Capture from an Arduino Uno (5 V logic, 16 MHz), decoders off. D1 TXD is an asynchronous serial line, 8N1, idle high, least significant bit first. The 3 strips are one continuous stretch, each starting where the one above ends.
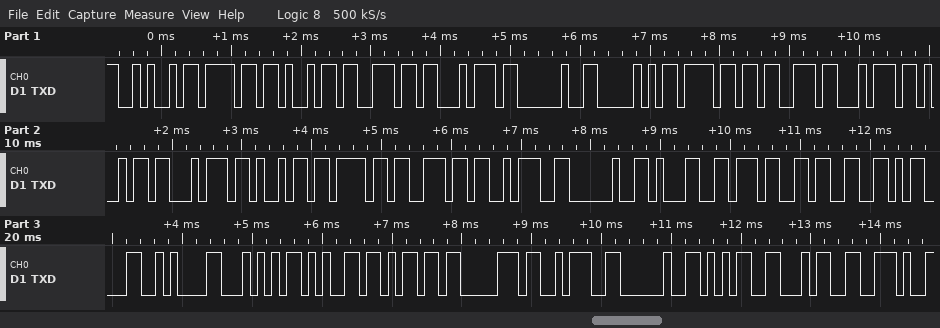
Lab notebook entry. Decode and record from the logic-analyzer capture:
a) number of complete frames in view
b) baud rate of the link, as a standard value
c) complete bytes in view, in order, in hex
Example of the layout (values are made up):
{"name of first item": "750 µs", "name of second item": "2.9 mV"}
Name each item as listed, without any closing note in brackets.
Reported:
{"number of complete frames in view": "31", "baud rate of the link, as a standard value": "9600 baud", "complete bytes in view, in order, in hex": "0x4A 0x6F 0x69 0x6E 0x74 0x20 0x50 0x6F 0x73 0x74 0x69 0x74 0x69 0x6F 0x6E 0x3A 0x20 0x31 0x37 0x33 0x0D 0x0A 0x54 0x65 0x6D 0x70 0x3A 0x20 0x35 0x34 0x2E"}
